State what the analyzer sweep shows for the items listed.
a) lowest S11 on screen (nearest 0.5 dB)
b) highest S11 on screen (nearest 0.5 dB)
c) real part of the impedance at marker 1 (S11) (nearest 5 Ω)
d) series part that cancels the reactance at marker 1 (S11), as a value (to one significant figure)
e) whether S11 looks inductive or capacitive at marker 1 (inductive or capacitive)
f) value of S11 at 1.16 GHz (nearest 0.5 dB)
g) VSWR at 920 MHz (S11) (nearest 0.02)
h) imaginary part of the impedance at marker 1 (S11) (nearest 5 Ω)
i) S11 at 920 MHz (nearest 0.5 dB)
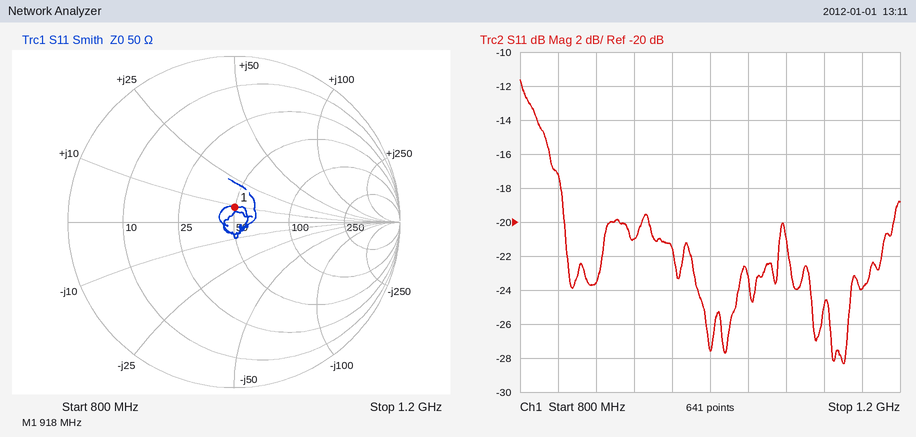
-28.5 dB
-11.5 dB
50 Ω
20 pF
inductive
-24.0 dB
1.20
+10 Ω
-21.0 dB
